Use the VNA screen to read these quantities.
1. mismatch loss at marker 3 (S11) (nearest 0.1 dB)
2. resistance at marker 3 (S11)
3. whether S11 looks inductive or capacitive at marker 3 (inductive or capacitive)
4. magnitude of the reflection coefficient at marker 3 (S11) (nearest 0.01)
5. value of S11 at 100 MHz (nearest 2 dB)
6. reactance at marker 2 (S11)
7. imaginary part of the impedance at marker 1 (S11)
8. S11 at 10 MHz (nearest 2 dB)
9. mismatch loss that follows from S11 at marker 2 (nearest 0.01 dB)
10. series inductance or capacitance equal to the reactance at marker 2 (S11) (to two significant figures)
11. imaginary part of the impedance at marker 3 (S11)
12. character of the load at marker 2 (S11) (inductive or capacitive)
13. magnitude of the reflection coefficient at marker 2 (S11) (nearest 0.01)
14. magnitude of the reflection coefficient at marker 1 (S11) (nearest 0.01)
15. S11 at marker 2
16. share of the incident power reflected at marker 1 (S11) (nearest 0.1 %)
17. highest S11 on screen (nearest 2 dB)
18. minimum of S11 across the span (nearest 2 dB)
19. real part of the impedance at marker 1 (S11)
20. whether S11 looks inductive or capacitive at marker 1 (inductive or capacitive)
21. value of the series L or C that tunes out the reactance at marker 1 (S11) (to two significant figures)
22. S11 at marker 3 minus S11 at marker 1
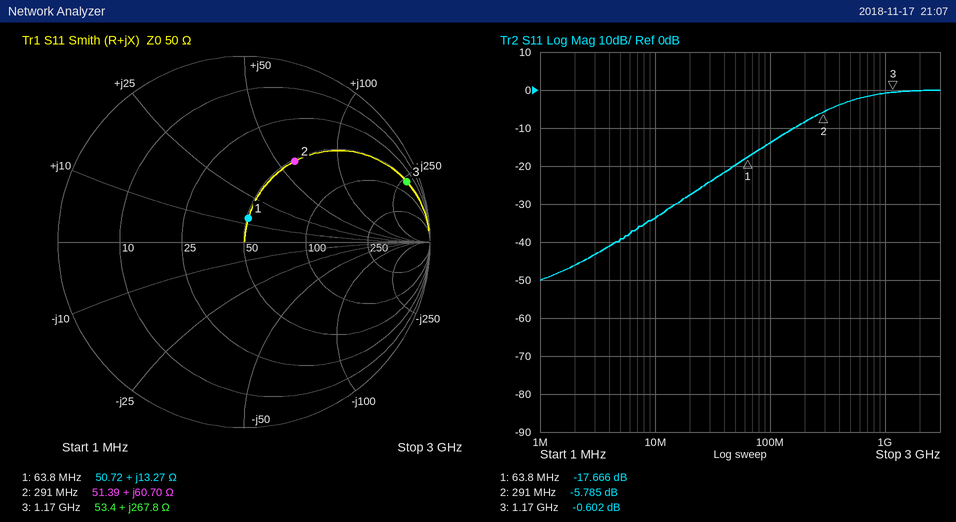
8.9 dB
53.4 Ω
inductive
0.93
-14 dB
+60.70 Ω
+13.27 Ω
-34 dB
1.33 dB
33 nH
+267.8 Ω
inductive
0.51
0.13
-5.785 dB
1.7 %
0 dB
-50 dB
50.72 Ω
inductive
190 pF
17.064 dB
